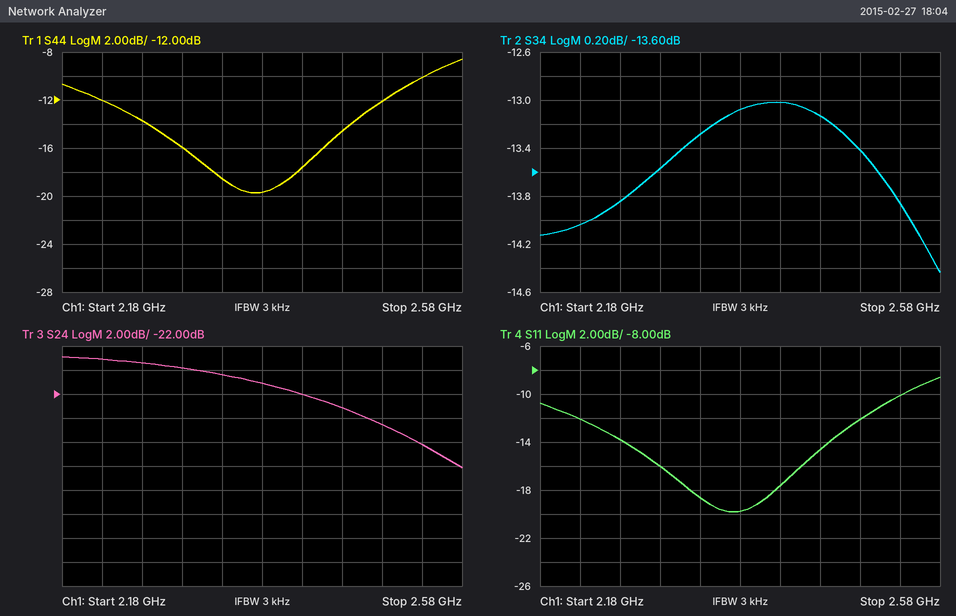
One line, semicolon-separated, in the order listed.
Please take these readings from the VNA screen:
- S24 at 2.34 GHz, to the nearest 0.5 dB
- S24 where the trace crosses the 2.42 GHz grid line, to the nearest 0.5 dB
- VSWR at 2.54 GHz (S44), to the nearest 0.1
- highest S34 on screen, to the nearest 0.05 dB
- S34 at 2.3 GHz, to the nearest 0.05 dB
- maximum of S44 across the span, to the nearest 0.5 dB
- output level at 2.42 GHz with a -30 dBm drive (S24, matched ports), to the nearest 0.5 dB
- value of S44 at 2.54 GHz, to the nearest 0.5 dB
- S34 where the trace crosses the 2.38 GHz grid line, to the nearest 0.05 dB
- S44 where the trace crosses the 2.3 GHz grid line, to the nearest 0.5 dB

-20.5 dB; -22.0 dB; 1.9; -13.00 dB; -13.55 dB; -8.5 dB; -52.0 dBm; -10.0 dB; -13.10 dB; -16.0 dB
